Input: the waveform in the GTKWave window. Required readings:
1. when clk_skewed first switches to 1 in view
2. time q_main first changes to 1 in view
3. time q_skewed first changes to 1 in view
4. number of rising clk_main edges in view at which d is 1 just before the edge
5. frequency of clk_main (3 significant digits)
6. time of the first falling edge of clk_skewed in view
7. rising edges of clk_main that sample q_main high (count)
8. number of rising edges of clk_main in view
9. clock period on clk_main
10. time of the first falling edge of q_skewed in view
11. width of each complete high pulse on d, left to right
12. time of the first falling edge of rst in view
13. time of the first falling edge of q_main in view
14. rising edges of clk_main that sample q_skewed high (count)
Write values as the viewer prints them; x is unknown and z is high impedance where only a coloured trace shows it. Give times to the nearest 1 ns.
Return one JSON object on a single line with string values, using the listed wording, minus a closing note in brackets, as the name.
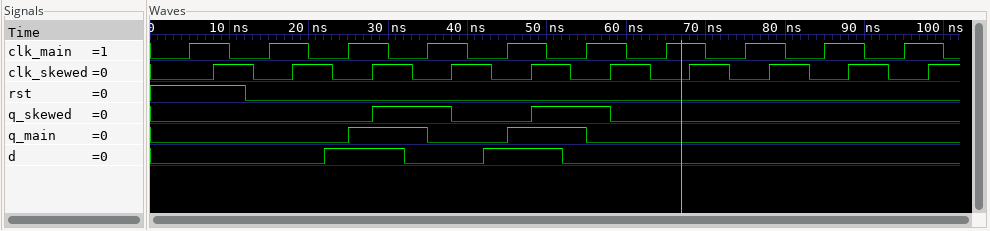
{"when clk_skewed first switches to 1 in view": "8 ns", "time q_main first changes to 1 in view": "25 ns", "time q_skewed first changes to 1 in view": "28 ns", "number of rising clk_main edges in view at which d is 1 just before the edge": "2", "frequency of clk_main": "100 MHz", "time of the first falling edge of clk_skewed in view": "13 ns", "rising edges of clk_main that sample q_main high": "2", "number of rising edges of clk_main in view": "10", "clock period on clk_main": "10 ns", "time of the first falling edge of q_skewed in view": "38 ns", "width of each complete high pulse on d, left to right": "10 ns, 10 ns", "time of the first falling edge of rst in view": "12 ns", "time of the first falling edge of q_main in view": "35 ns", "rising edges of clk_main that sample q_skewed high": "2"}
